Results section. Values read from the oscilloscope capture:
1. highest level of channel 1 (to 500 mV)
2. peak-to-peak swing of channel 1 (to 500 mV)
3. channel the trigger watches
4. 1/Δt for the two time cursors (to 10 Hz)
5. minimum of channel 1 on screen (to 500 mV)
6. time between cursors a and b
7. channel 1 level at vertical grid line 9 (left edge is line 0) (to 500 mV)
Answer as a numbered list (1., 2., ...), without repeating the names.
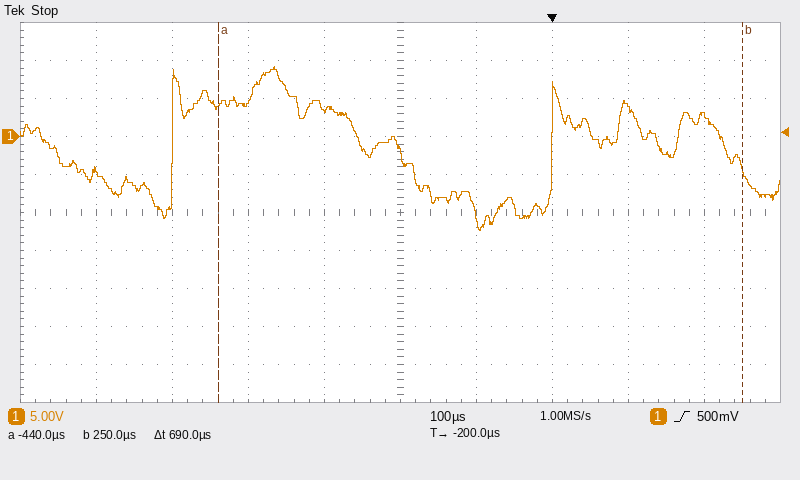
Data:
1. 9.0 V
2. 21.5 V
3. channel 1
4. 1.45 kHz
5. -12.5 V
6. 690 µs
7. 3.0 V
